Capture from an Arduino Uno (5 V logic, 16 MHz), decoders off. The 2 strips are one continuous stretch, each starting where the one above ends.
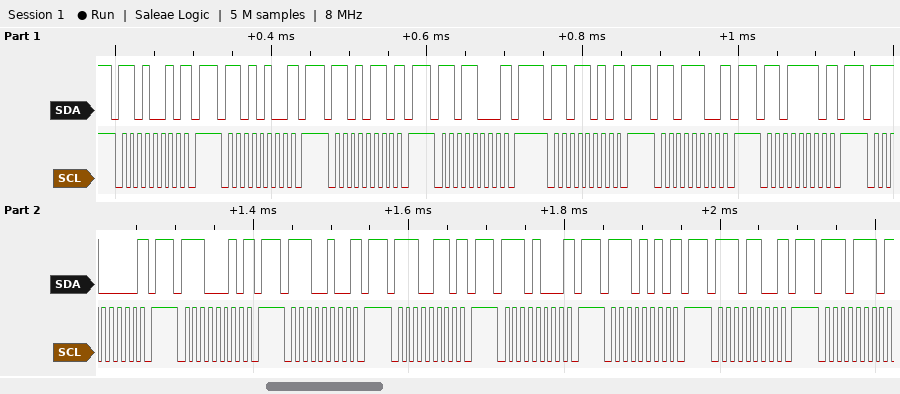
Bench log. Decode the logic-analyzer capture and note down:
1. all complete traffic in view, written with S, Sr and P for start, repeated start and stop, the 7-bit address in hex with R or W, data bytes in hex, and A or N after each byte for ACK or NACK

S 69W N P S 6AW N P S 6BW N P S 6CW N P S 6DW N P S 6EW N P S 6FW N P S 70W N P S 71W N P S 72W N P S 73W N P S 74W N P S 75W N P S 76W N P S 77W N
